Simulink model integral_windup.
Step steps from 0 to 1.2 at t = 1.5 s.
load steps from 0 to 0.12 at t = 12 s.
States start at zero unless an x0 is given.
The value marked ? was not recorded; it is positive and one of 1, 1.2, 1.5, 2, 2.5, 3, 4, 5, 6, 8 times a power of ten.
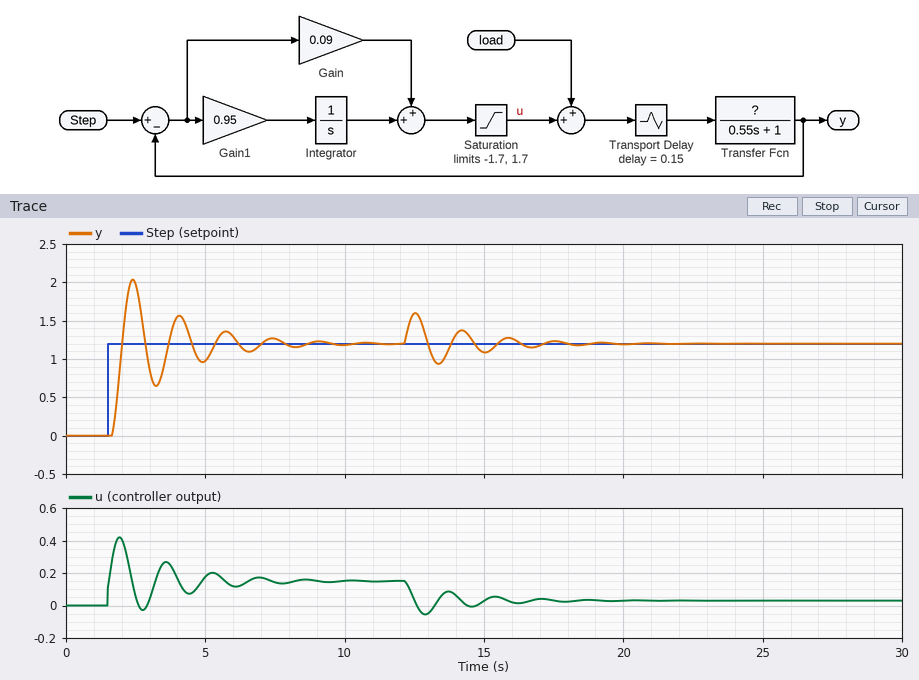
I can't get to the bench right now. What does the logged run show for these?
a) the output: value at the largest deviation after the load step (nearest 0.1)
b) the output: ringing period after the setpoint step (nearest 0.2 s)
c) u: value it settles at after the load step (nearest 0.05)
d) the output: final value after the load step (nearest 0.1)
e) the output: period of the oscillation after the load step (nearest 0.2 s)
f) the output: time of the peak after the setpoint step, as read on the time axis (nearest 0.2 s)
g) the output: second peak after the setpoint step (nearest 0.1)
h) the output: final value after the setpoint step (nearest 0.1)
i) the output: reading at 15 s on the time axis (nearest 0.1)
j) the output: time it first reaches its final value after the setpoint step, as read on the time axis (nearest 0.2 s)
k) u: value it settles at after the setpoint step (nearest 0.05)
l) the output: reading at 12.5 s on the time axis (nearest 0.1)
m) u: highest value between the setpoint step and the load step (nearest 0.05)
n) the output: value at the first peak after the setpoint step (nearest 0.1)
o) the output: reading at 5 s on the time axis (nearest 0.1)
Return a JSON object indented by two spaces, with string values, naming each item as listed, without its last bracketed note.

{
  "the output: value at the largest deviation after the load step": "1.6",
  "the output: ringing period after the setpoint step": "1.6 s",
  "u: value it settles at after the load step": "0.05",
  "the output: final value after the load step": "1.2",
  "the output: period of the oscillation after the load step": "1.6 s",
  "the output: time of the peak after the setpoint step, as read on the time axis": "2.4 s",
  "the output: second peak after the setpoint step": "1.6",
  "the output: final value after the setpoint step": "1.2",
  "the output: reading at 15 s on the time axis": "1.1",
  "the output: time it first reaches its final value after the setpoint step, as read on the time axis": "2.0 s",
  "u: value it settles at after the setpoint step": "0.15",
  "the output: reading at 12.5 s on the time axis": "1.6",
  "u: highest value between the setpoint step and the load step": "0.40",
  "the output: value at the first peak after the setpoint step": "2.0",
  "the output: reading at 5 s on the time axis": "1.0"
}
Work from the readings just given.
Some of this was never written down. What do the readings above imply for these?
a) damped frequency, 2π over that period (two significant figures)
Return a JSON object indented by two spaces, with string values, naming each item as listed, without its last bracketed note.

{
  "damped frequency, 2π over that period": "3.9 rad/s"
}
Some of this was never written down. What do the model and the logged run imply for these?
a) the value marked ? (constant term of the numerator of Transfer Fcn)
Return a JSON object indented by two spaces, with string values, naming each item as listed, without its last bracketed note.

{
  "the value marked ?": "8"
}
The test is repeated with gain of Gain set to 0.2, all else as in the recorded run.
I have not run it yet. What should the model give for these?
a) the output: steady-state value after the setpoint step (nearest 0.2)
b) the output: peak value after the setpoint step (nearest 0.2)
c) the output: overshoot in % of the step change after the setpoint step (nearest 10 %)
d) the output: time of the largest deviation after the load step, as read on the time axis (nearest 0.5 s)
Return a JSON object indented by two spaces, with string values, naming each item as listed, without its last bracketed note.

{
  "the output: steady-state value after the setpoint step": "1.2",
  "the output: peak value after the setpoint step": "1.8",
  "the output: overshoot in % of the step change after the setpoint step": "50 %",
  "the output: time of the largest deviation after the load step, as read on the time axis": "12.5 s"
}
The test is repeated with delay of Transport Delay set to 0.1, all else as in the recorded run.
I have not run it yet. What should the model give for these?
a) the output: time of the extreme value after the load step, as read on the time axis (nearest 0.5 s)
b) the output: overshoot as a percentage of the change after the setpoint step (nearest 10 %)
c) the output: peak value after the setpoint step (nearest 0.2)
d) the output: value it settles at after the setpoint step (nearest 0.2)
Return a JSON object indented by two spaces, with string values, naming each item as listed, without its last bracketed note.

{
  "the output: time of the extreme value after the load step, as read on the time axis": "12.5 s",
  "the output: overshoot as a percentage of the change after the setpoint step": "50 %",
  "the output: peak value after the setpoint step": "1.8",
  "the output: value it settles at after the setpoint step": "1.2"
}
